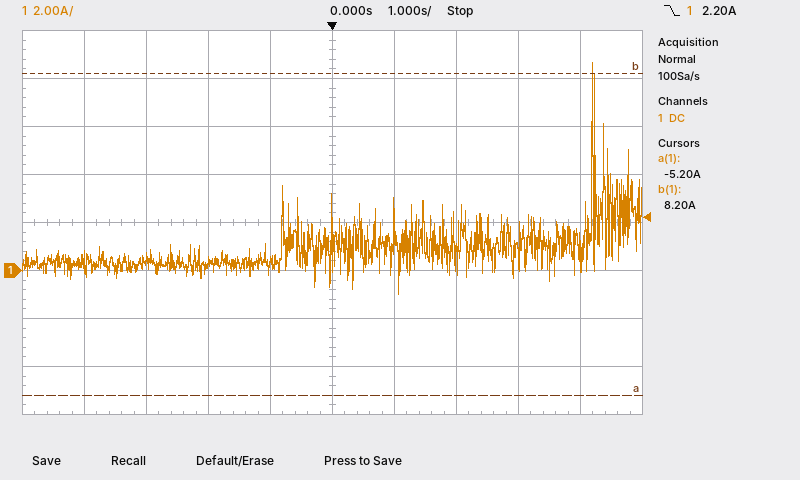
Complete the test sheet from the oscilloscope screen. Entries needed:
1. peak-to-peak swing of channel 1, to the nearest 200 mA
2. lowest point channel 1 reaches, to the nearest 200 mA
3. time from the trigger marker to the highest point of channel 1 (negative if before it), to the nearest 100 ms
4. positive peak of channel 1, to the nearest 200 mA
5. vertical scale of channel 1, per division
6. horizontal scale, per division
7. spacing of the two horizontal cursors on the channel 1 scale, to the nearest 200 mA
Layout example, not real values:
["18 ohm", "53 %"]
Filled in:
["9.6 A", "-1.0 A", "+4.2 s", "8.6 A", "2 A", "1 s", "13.4 A"]
